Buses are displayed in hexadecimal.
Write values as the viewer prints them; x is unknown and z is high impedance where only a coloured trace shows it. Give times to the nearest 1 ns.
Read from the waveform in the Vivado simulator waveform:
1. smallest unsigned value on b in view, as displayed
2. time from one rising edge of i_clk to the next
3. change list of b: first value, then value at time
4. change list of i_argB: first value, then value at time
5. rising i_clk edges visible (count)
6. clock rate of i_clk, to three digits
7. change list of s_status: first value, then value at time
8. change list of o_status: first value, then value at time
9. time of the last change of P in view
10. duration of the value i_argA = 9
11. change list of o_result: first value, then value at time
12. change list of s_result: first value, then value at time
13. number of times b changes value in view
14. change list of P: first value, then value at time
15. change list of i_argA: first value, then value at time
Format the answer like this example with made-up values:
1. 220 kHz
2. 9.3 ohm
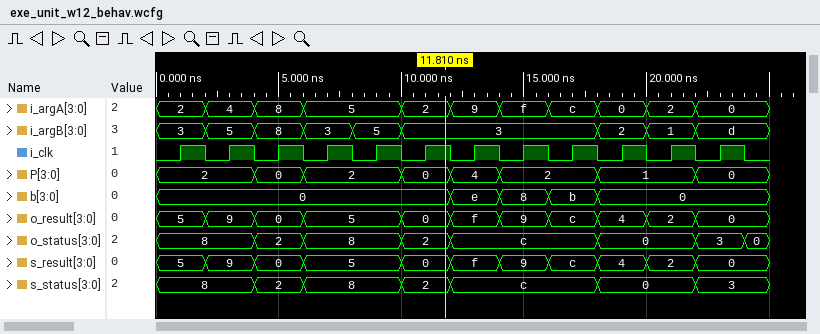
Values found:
1. 0
2. 2 ns
3. 0, e at 12 ns, 8 at 14 ns, b at 16 ns, 0 at 18 ns
4. 3, 5 at 2 ns, 8 at 4 ns, 3 at 6 ns, 5 at 8 ns, 3 at 10 ns, 2 at 18 ns, 1 at 20 ns, d at 22 ns
5. 12
6. 500 MHz
7. 8, 2 at 4 ns, 8 at 6 ns, 2 at 10 ns, c at 12 ns, 0 at 18 ns, 3 at 22 ns
8. 8, 2 at 4 ns, 8 at 6 ns, 2 at 10 ns, c at 12 ns, 0 at 18 ns, 3 at 22 ns, 0 at 24 ns
9. 22 ns
10. 2 ns
11. 5, 9 at 2 ns, 0 at 4 ns, 5 at 6 ns, 0 at 10 ns, f at 12 ns, 9 at 14 ns, c at 16 ns, 4 at 18 ns, 2 at 20 ns, 0 at 22 ns
12. 5, 9 at 2 ns, 0 at 4 ns, 5 at 6 ns, 0 at 10 ns, f at 12 ns, 9 at 14 ns, c at 16 ns, 4 at 18 ns, 2 at 20 ns, 0 at 22 ns
13. 4
14. 2, 0 at 4 ns, 2 at 6 ns, 0 at 10 ns, 4 at 12 ns, 2 at 14 ns, 1 at 18 ns, 0 at 22 ns
15. 2, 4 at 2 ns, 8 at 4 ns, 5 at 6 ns, 2 at 10 ns, 9 at 12 ns, f at 14 ns, c at 16 ns, 0 at 18 ns, 2 at 20 ns, 0 at 22 ns
